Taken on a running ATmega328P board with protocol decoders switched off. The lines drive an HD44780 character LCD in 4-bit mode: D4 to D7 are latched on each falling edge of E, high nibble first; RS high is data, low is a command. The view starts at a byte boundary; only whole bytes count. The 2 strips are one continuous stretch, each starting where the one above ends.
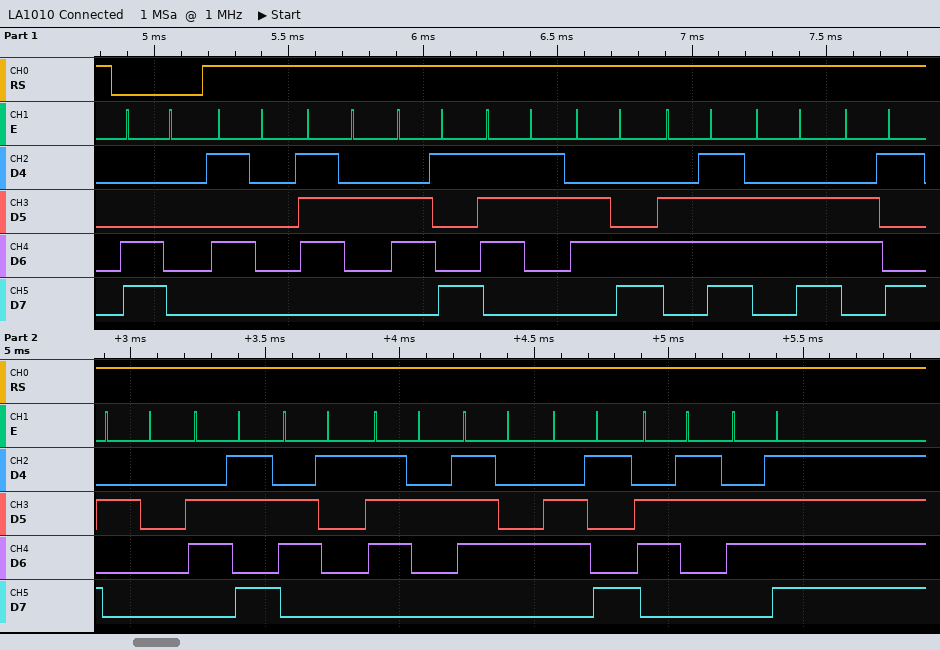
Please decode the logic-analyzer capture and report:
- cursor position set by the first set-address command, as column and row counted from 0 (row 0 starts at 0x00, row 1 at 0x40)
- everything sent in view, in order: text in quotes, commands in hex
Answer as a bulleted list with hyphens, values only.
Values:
- column 0, row 1
- 0xC0 "Prisloni kartico"
